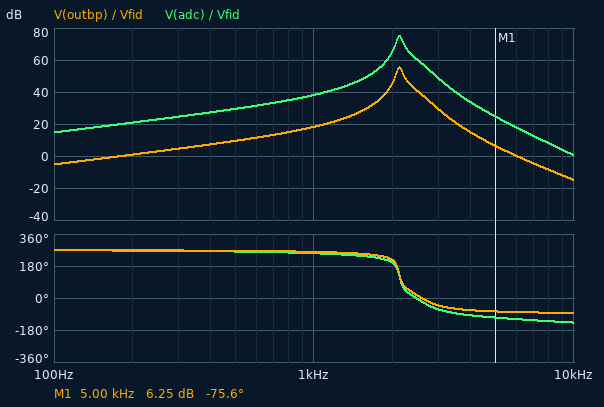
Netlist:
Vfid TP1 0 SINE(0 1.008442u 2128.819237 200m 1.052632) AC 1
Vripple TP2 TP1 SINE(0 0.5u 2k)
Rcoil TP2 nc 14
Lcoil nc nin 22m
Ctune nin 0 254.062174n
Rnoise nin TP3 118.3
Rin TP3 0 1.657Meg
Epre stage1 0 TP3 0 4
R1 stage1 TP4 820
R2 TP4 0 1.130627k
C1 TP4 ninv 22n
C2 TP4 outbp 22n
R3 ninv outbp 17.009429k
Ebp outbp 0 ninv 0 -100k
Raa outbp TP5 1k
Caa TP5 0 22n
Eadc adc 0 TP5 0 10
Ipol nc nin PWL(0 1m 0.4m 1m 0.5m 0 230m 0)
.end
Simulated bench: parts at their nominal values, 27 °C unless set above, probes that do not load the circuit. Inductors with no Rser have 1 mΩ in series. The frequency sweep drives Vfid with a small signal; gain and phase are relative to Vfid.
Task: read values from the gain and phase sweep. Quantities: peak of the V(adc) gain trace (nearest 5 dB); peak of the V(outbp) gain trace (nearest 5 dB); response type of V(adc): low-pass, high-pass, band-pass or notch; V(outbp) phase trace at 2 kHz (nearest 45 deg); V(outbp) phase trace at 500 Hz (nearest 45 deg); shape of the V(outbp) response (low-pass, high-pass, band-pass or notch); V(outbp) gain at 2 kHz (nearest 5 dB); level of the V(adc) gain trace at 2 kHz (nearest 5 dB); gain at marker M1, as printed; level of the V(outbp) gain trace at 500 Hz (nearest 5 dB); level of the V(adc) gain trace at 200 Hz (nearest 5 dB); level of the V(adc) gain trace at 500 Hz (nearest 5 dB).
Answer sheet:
75 dB
55 dB
band-pass
225 deg
270 deg
band-pass
45 dB
65 dB
6.25 dB
10 dB
20 dB
30 dB
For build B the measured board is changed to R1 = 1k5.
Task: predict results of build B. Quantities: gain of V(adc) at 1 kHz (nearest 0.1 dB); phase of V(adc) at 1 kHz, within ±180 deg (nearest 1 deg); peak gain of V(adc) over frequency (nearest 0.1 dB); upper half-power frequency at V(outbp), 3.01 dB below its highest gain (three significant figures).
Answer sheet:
36.0 dB
-112 deg
73.1 dB
2.18 kHz
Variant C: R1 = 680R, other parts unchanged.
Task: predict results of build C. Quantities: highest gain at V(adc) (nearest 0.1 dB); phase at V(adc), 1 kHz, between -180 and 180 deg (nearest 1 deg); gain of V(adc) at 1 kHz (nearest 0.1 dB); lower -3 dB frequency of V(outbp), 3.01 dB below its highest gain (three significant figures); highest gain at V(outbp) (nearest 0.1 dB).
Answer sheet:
74.9 dB
-107 deg
38.7 dB
2.08 kHz
55.3 dB
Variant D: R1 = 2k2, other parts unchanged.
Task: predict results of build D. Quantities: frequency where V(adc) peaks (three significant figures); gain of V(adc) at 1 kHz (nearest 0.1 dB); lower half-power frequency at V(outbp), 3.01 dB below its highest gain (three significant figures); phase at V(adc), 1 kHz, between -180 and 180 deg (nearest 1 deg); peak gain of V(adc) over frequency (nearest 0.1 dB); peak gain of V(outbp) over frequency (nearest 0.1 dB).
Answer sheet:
2.13 kHz
34.3 dB
2.07 kHz
-115 deg
69.6 dB
50.0 dB
